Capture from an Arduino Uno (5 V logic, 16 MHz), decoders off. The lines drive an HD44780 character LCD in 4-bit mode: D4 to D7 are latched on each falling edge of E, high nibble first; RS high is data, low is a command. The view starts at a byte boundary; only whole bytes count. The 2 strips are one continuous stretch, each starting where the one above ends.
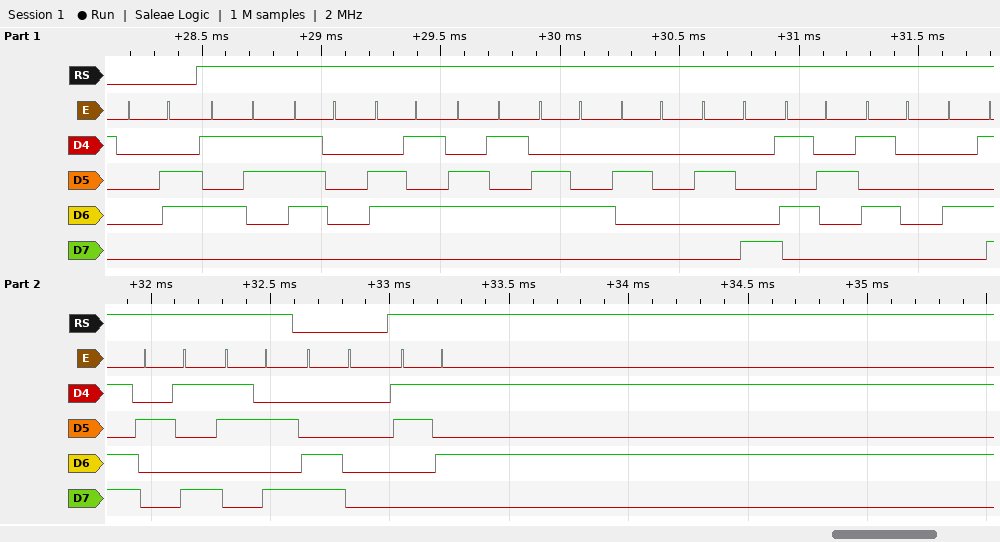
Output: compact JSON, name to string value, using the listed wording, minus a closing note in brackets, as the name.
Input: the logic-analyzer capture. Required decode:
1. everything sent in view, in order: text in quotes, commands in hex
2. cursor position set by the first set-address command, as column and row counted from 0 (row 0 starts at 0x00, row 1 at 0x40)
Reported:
{"everything sent in view, in order: text in quotes, commands in hex": "0x06 \"Speed (RPM):\" 0xC0 \"5\"", "cursor position set by the first set-address command, as column and row counted from 0": "column 0, row 1"}
